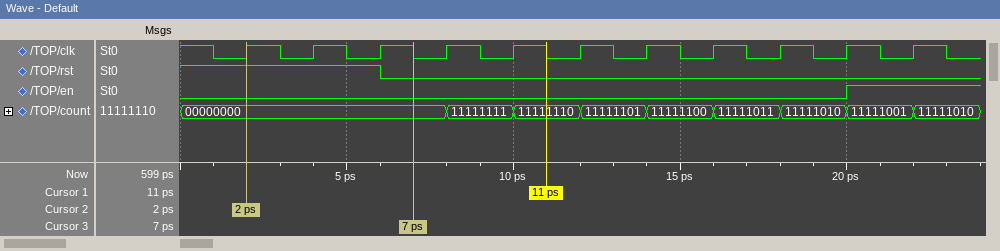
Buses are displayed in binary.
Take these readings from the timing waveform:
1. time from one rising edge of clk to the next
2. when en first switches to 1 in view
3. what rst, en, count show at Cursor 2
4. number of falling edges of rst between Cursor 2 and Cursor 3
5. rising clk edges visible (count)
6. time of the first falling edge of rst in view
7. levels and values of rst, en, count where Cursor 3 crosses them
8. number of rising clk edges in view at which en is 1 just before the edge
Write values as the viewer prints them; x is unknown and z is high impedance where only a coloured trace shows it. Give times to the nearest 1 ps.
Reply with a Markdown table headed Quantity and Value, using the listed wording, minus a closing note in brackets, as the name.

| Quantity | Value |
|---|---|
| time from one rising edge of clk to the next | 2 ps |
| when en first switches to 1 in view | 20 ps |
| what rst, en, count show at Cursor 2 | rst=1, en=0, count=00000000 |
| number of falling edges of rst between Cursor 2 and Cursor 3 | 1 |
| rising clk edges visible | 11 |
| time of the first falling edge of rst in view | 6 ps |
| levels and values of rst, en, count where Cursor 3 crosses them | rst=0, en=0, count=00000000 |
| number of rising clk edges in view at which en is 1 just before the edge | 1 |
